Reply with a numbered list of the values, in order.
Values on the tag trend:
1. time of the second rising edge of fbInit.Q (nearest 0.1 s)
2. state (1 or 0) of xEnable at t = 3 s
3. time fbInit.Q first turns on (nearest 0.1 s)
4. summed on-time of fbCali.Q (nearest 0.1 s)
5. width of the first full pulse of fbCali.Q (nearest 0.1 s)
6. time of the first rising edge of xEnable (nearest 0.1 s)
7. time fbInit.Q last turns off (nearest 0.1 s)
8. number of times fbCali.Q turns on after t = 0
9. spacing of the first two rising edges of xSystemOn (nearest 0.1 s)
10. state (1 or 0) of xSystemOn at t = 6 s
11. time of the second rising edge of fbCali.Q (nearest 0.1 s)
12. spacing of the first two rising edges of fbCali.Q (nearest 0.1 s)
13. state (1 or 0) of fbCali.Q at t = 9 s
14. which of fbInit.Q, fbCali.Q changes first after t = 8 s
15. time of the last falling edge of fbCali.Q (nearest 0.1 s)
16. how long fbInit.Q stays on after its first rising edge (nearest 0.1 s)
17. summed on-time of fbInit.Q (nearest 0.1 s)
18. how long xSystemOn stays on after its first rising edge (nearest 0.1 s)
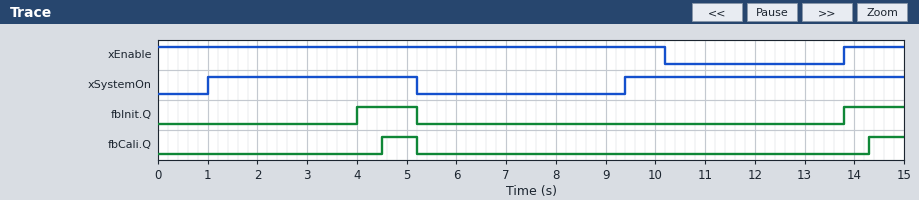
1. 13.8 s
2. 1
3. 4.0 s
4. 1.4 s
5. 0.7 s
6. 13.8 s
7. 5.2 s
8. 2
9. 8.4 s
10. 0
11. 14.3 s
12. 9.8 s
13. 0
14. fbInit.Q
15. 5.2 s
16. 1.2 s
17. 2.4 s
18. 4.2 s
